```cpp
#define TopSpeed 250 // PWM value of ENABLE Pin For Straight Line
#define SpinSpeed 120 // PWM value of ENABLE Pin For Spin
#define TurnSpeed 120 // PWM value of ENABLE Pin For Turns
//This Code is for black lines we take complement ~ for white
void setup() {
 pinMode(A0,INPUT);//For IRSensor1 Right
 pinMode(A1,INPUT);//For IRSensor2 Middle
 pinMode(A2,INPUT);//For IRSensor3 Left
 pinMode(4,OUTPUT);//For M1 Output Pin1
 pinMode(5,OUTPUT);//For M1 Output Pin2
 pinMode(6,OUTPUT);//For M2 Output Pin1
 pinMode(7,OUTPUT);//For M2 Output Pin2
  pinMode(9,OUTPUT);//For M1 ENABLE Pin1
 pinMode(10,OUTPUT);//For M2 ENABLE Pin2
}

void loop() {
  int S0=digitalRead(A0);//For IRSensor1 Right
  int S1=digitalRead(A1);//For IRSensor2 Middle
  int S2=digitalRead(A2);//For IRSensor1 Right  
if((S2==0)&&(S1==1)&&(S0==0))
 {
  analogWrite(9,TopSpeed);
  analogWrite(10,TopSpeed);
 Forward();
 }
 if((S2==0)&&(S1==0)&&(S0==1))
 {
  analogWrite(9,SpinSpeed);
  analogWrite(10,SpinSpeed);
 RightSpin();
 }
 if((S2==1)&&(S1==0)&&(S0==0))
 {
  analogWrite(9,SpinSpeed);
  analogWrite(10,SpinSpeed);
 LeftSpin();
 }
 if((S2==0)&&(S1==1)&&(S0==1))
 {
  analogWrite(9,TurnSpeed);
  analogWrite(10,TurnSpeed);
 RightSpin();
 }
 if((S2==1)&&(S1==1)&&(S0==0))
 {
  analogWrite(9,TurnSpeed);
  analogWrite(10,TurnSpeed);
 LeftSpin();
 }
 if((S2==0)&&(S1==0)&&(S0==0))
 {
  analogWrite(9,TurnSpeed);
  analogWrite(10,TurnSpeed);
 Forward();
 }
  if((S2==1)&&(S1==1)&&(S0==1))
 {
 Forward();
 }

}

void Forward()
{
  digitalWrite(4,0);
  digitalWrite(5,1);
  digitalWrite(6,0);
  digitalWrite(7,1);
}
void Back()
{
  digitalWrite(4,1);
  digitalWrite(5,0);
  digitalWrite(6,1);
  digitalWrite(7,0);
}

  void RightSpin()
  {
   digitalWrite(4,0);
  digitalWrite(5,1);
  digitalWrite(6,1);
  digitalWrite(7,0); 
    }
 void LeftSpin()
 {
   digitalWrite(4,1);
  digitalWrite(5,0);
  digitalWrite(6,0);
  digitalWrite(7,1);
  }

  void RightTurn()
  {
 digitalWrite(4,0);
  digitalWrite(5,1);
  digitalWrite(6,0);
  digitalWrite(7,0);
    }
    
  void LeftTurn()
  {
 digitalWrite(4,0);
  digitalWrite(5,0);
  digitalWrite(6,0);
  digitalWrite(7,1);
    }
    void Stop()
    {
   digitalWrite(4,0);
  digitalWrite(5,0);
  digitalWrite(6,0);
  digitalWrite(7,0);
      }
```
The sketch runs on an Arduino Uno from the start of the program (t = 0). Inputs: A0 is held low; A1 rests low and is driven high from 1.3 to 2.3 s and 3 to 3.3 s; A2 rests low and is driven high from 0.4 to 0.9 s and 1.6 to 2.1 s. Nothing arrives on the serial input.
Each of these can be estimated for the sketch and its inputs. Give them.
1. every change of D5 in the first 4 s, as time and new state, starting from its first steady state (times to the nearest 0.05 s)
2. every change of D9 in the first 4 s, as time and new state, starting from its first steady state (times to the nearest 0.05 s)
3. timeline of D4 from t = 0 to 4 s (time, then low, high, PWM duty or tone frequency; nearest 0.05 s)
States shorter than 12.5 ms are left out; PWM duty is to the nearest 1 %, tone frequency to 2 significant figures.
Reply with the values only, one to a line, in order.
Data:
0 s high; 0.4 s low; 0.9 s high; 1.6 s low; 2.1 s high
0 s PWM 47 %; 1.3 s PWM 98 %; 1.6 s PWM 47 %; 2.1 s PWM 98 %; 2.3 s PWM 47 %; 3 s PWM 98 %; 3.3 s PWM 47 %
0 s low; 0.4 s high; 0.9 s low; 1.6 s high; 2.1 s low
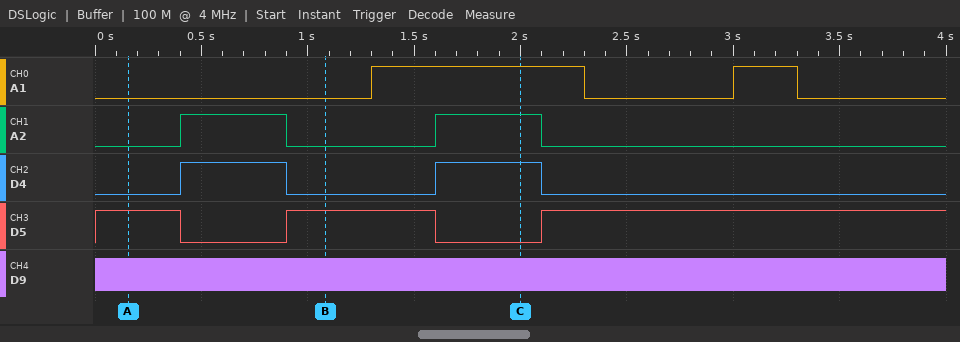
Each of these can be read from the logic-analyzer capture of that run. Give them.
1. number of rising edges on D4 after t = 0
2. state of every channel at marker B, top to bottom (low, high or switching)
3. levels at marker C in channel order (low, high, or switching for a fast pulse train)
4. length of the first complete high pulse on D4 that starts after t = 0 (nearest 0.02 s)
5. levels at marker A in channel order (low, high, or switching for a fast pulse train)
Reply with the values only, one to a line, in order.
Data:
2
A1 low, A2 low, D4 low, D5 high, D9 switching
A1 high, A2 high, D4 high, D5 low, D9 switching
0.50 s
A1 low, A2 low, D4 low, D5 high, D9 switching
